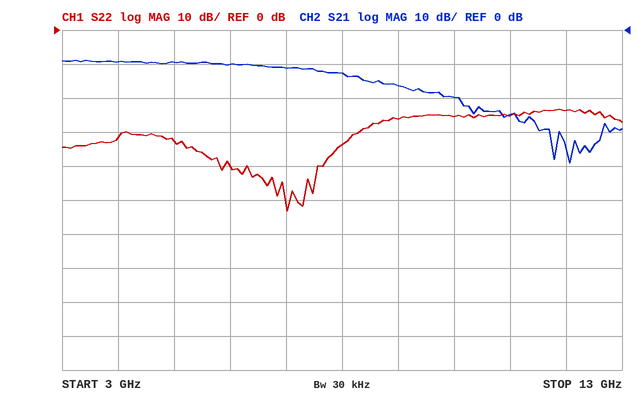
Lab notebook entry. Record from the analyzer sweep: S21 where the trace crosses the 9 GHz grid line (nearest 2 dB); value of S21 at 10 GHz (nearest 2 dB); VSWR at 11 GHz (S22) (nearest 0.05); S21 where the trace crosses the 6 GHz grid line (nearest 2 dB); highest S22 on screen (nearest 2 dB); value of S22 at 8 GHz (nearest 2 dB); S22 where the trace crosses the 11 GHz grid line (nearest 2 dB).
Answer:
-16 dB
-20 dB
1.10
-10 dB
-24 dB
-34 dB
-26 dB
